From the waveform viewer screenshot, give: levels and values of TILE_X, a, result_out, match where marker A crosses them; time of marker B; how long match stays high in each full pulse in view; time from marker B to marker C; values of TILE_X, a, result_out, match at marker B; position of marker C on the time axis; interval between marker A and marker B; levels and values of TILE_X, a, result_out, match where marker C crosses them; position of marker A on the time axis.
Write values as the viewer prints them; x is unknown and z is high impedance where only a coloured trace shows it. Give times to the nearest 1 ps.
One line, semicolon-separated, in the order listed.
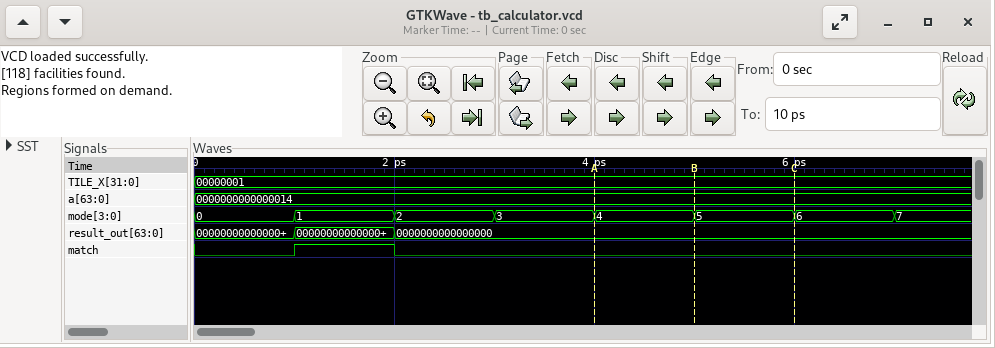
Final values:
TILE_X=00000001, a=0000000000000014, result_out=0000000000000000, match=0; 5 ps; 1 ps; 1 ps; TILE_X=00000001, a=0000000000000014, result_out=0000000000000000, match=0; 6 ps; 1 ps; TILE_X=00000001, a=0000000000000014, result_out=0000000000000000, match=0; 4 ps
